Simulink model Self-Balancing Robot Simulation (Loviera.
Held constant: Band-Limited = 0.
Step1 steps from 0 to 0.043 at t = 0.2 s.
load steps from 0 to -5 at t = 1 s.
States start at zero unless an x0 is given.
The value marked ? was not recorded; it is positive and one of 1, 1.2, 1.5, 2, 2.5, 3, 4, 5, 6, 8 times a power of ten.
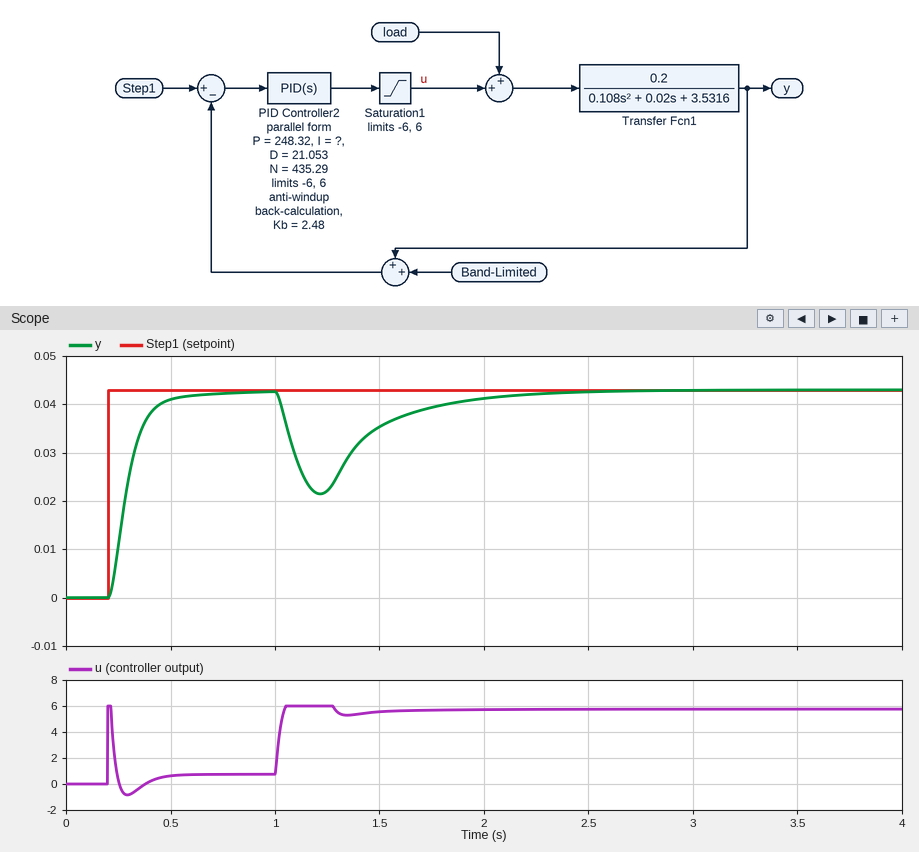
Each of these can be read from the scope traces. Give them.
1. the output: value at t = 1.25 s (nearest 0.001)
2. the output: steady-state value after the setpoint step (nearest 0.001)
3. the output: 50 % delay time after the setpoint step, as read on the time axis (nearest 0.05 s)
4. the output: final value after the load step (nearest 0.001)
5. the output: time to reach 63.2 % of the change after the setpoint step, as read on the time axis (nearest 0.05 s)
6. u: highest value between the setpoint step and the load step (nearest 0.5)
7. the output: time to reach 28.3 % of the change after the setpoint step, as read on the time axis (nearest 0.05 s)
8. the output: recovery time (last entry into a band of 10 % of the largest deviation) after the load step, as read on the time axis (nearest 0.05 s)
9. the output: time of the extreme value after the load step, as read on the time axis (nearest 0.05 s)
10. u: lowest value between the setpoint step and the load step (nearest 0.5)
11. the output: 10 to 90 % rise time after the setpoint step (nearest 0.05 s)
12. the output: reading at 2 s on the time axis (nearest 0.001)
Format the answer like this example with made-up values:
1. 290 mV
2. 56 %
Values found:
1. 0.022
2. 0.043
3. 0.30 s
4. 0.043
5. 0.30 s
6. 6.0
7. 0.25 s
8. 1.95 s
9. 1.20 s
10. -1.0
11. 0.20 s
12. 0.041
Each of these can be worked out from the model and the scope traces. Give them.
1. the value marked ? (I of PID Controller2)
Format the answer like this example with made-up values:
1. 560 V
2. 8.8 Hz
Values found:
1. 600
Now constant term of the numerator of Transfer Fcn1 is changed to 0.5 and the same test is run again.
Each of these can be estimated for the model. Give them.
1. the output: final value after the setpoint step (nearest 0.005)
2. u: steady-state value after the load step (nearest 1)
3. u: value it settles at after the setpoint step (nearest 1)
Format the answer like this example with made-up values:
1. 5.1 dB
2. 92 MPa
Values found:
1. 0.045
2. 5
3. 0
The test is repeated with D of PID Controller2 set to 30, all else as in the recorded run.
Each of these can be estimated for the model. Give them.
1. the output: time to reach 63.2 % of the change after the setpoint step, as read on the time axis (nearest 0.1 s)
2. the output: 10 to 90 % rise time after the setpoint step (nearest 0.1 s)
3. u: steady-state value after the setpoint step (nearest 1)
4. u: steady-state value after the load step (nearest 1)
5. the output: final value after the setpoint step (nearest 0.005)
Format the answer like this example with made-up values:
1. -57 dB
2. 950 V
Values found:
1. 0.4 s
2. 0.3 s
3. 1
4. 6
5. 0.045
